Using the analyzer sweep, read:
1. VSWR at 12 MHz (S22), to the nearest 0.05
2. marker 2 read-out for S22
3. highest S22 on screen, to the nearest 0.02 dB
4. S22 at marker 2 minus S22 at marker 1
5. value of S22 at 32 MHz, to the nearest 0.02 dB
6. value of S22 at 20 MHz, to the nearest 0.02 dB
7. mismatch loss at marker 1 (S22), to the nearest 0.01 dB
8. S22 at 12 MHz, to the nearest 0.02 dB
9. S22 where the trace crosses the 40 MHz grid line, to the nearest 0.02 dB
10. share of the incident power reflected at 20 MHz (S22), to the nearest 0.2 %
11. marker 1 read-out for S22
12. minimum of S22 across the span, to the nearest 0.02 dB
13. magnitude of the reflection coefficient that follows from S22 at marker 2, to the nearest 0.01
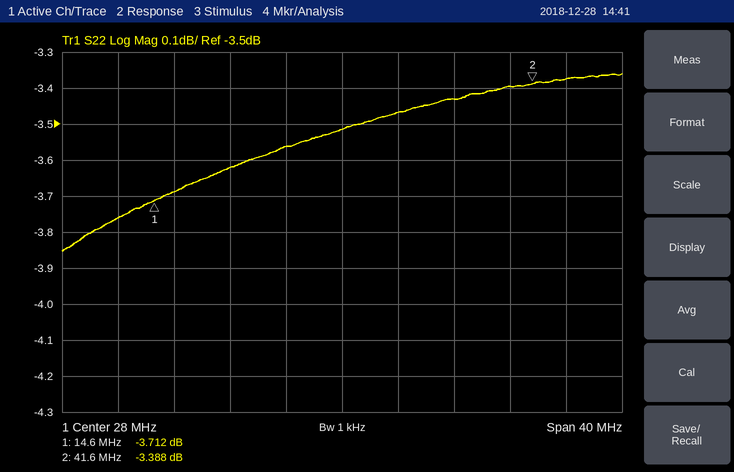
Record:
4.70
-3.388 dB
-3.36 dB
0.324 dB
-3.46 dB
-3.62 dB
2.41 dB
-3.76 dB
-3.40 dB
43.4 %
-3.712 dB
-3.86 dB
0.68
